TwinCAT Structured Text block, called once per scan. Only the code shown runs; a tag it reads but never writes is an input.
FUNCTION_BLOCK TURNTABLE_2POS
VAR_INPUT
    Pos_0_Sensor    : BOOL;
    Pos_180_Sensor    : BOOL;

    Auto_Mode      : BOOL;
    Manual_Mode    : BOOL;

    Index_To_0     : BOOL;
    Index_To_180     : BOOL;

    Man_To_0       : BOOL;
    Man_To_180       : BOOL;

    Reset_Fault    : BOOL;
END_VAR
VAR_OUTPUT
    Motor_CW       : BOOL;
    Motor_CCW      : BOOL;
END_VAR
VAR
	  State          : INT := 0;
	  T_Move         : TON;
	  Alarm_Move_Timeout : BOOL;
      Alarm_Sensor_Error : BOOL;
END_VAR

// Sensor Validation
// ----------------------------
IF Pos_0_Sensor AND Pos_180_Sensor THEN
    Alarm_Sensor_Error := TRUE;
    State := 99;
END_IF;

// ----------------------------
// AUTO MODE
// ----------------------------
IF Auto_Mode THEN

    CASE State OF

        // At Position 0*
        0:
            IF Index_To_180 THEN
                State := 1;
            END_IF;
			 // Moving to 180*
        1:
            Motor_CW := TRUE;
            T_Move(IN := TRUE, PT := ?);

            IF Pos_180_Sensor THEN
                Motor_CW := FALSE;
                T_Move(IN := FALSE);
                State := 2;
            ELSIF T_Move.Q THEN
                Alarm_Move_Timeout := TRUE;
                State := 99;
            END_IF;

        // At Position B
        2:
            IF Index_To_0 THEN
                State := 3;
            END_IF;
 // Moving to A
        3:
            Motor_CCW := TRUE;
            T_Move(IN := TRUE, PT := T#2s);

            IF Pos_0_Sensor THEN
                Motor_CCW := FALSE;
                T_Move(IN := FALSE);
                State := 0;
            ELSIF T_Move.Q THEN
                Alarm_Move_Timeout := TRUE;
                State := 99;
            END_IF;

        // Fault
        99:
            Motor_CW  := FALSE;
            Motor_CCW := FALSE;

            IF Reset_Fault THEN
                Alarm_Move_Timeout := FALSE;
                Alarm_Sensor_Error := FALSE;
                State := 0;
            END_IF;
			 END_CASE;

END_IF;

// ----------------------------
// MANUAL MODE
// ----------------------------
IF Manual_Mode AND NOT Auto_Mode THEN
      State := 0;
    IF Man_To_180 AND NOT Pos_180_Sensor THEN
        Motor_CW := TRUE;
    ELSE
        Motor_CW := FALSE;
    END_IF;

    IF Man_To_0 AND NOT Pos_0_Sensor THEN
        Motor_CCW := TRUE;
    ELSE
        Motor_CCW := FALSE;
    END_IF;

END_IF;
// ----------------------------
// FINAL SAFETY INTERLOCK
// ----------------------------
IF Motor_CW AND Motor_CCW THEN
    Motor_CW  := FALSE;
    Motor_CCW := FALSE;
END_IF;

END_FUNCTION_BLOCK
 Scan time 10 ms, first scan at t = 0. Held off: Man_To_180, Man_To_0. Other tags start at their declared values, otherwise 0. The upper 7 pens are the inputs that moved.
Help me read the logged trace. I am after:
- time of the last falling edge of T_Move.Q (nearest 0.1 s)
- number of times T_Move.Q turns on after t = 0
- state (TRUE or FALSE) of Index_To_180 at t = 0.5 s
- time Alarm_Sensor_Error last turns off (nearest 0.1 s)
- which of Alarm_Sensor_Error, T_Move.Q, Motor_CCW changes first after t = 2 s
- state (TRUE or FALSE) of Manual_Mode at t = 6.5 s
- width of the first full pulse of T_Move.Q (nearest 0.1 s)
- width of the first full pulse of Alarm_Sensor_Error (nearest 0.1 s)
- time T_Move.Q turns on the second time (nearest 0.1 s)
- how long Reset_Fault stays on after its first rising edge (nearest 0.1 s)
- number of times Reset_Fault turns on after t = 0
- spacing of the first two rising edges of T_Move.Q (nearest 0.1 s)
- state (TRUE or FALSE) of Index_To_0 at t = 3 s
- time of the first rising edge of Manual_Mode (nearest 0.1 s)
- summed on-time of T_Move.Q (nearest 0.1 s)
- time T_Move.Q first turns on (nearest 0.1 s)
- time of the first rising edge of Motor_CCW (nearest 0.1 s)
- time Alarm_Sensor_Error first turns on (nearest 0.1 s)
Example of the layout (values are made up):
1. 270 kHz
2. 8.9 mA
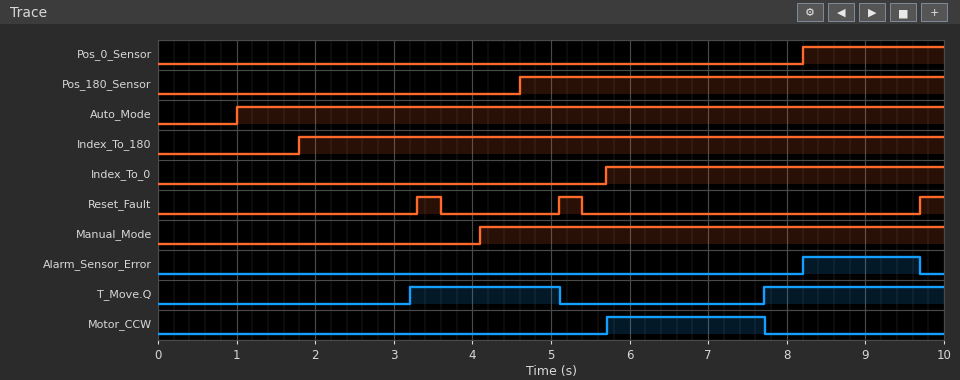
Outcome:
1. 5.1 s
2. 2
3. FALSE
4. 9.7 s
5. T_Move.Q
6. TRUE
7. 1.9 s
8. 1.5 s
9. 7.7 s
10. 0.3 s
11. 3
12. 4.5 s
13. FALSE
14. 4.1 s
15. 4.2 s
16. 3.2 s
17. 5.7 s
18. 8.2 s
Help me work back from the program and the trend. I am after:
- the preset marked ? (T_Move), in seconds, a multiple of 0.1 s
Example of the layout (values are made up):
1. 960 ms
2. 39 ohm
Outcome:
1. 1.4 s
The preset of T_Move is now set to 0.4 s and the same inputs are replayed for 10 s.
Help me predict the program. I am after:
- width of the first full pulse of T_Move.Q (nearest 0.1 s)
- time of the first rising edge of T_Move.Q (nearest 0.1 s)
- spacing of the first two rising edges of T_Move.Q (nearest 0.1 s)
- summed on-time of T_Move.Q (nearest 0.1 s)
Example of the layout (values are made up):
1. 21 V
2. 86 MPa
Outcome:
1. 2.9 s
2. 2.2 s
3. 5.5 s
4. 5.2 s
